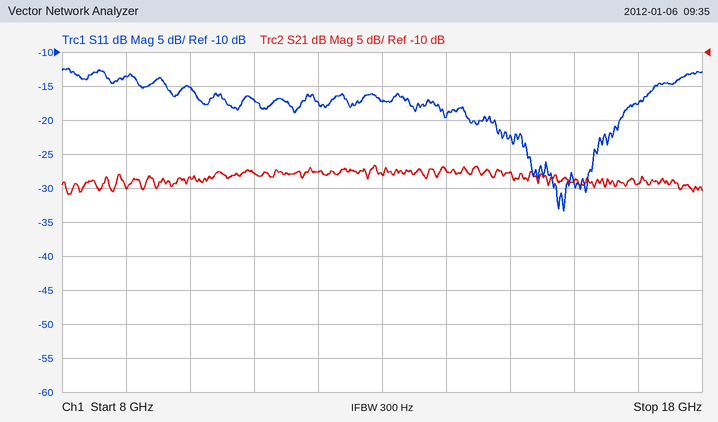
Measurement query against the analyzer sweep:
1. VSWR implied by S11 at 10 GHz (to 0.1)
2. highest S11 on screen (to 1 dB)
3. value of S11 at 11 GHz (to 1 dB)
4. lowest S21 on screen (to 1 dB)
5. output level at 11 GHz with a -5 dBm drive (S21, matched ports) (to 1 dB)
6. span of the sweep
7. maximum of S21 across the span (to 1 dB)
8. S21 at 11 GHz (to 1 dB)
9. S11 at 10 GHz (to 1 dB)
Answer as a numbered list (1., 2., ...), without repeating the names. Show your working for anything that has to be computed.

1. |Γ| = 10^(-15/20) = 0.1778; VSWR = (1 + 0.1778)/(1 − 0.1778) ≈ 1.4
2. -12 dB
3. -17 dB
4. -31 dB
5. -5 dBm + (-28 dB) = -33 dBm
6. 10 GHz
7. -27 dB
8. -28 dB
9. -15 dB
